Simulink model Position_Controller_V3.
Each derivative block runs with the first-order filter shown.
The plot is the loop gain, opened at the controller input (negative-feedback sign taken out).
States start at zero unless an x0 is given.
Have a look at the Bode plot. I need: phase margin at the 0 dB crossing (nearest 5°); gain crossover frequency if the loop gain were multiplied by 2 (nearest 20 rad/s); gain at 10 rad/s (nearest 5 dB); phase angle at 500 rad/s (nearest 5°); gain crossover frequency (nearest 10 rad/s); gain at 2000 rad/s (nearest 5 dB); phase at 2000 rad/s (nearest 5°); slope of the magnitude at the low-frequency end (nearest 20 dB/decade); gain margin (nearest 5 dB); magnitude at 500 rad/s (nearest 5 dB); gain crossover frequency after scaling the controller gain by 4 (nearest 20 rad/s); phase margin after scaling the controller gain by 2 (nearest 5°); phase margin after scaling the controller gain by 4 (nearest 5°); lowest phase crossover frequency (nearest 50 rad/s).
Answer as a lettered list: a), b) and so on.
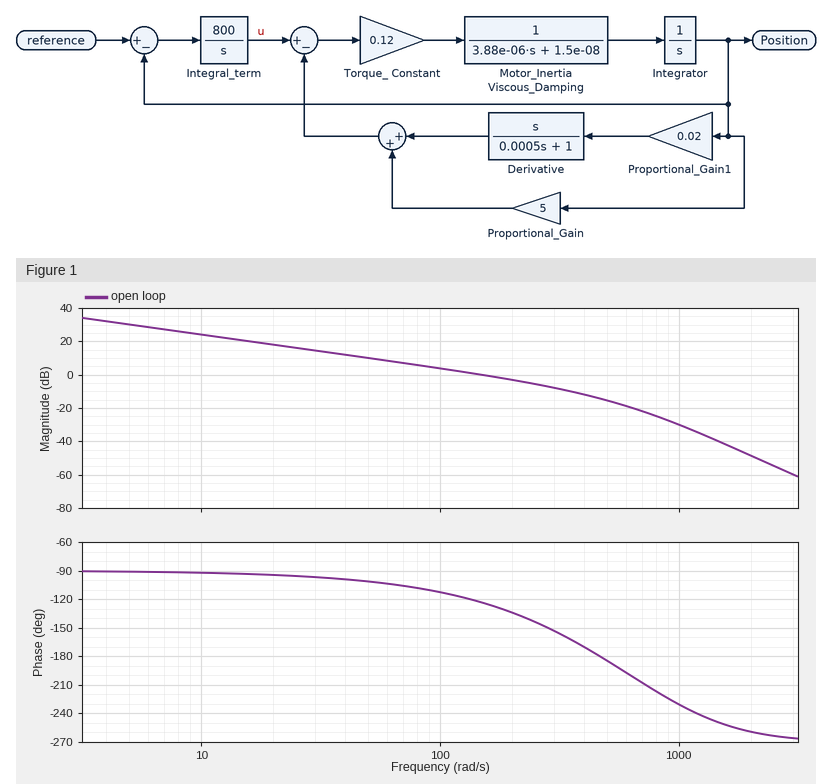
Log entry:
a) 55°
b) 260 rad/s
c) 25 dB
d) -185°
e) 150 rad/s
f) -50 dB
g) -260°
h) -20 dB/decade
i) 15 dB
j) -15 dB
k) 400 rad/s
l) 35°
m) 10°
n) 450 rad/s
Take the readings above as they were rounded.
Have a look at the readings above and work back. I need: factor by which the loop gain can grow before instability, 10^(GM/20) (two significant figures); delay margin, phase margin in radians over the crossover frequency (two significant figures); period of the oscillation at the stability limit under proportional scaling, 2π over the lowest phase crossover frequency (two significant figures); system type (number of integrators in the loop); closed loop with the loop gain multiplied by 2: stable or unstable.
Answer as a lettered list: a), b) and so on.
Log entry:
a) 5.6
b) 0.0064 s
c) 0.014 s
d) 1
e) stable
